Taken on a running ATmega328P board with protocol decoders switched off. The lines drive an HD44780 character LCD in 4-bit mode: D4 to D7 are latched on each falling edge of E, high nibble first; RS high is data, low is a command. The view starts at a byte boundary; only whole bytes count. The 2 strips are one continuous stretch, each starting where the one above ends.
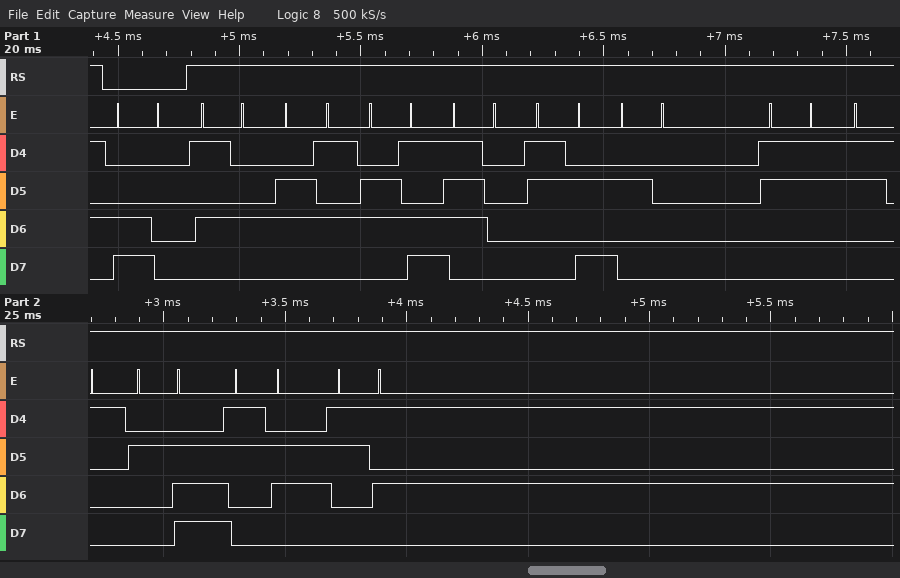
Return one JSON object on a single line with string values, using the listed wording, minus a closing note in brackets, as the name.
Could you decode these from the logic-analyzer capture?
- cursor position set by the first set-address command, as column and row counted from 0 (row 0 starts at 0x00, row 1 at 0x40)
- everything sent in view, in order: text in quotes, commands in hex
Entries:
{"cursor position set by the first set-address command, as column and row counted from 0": "column 0, row 1", "everything sent in view, in order: text in quotes, commands in hex": "0xC0 \"Temp: 31.65\""}
